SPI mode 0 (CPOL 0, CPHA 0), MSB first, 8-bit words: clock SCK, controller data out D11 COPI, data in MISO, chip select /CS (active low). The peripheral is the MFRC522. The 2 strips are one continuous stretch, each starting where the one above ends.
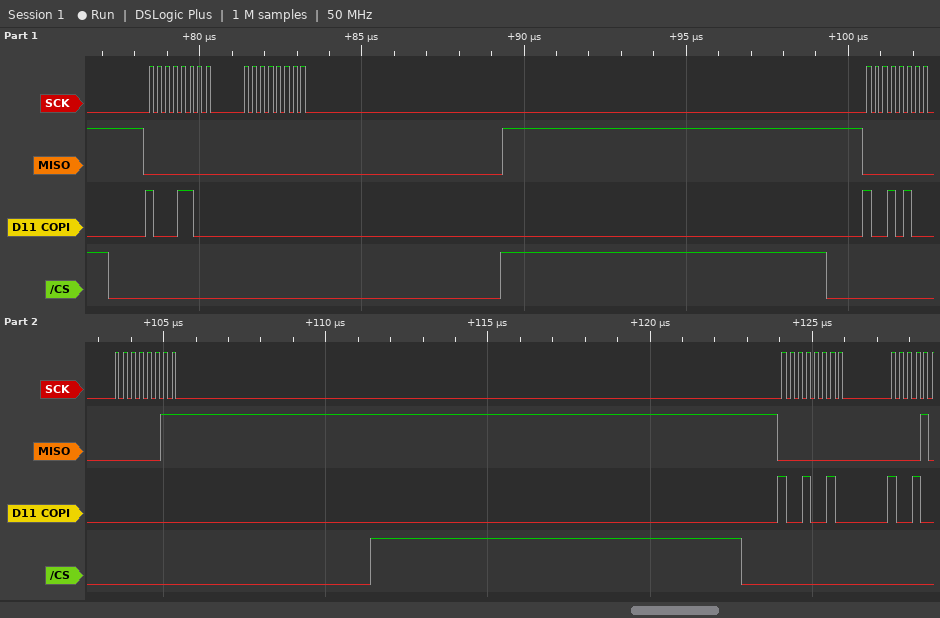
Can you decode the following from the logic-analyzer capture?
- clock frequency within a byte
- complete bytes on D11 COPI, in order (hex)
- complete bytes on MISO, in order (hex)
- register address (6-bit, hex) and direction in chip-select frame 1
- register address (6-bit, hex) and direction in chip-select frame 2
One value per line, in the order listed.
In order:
4 MHz
8C 00 94 00 92
00 00 00 03 00
0x06 read
0x0A read
